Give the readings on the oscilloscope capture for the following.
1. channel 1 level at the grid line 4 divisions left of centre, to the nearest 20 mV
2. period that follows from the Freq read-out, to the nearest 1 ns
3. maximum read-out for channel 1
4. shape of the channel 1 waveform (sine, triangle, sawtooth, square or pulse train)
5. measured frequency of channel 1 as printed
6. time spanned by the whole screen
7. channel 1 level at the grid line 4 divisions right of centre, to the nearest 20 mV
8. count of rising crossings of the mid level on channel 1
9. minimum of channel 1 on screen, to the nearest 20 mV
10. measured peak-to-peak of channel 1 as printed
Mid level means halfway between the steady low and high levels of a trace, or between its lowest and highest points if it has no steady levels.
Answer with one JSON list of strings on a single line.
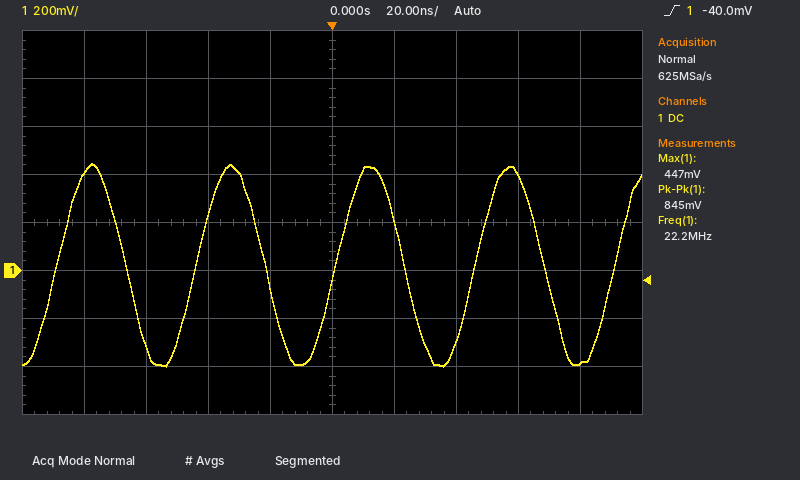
["400 mV", "45 ns", "447 mV", "sine", "22.2 MHz", "200 ns", "-380 mV", "5", "-400 mV", "845 mV"]
